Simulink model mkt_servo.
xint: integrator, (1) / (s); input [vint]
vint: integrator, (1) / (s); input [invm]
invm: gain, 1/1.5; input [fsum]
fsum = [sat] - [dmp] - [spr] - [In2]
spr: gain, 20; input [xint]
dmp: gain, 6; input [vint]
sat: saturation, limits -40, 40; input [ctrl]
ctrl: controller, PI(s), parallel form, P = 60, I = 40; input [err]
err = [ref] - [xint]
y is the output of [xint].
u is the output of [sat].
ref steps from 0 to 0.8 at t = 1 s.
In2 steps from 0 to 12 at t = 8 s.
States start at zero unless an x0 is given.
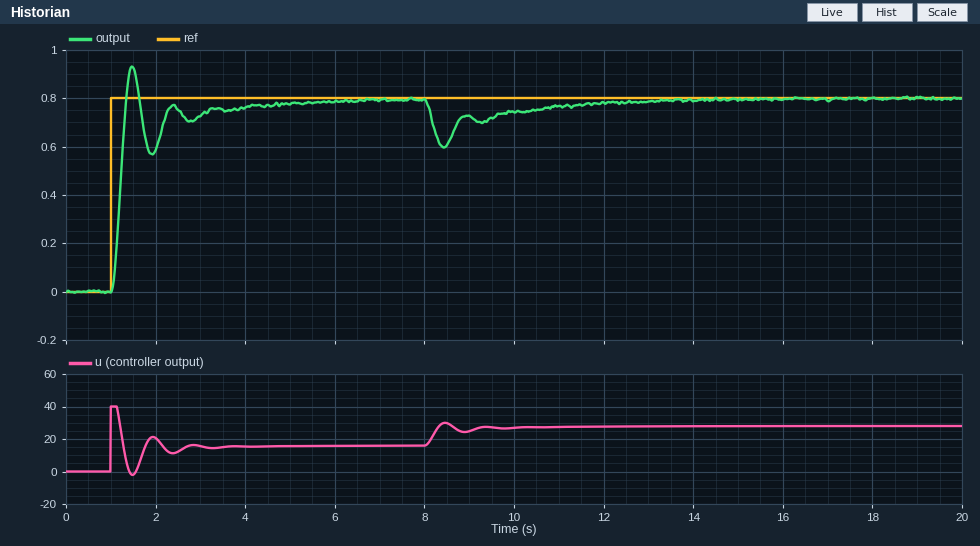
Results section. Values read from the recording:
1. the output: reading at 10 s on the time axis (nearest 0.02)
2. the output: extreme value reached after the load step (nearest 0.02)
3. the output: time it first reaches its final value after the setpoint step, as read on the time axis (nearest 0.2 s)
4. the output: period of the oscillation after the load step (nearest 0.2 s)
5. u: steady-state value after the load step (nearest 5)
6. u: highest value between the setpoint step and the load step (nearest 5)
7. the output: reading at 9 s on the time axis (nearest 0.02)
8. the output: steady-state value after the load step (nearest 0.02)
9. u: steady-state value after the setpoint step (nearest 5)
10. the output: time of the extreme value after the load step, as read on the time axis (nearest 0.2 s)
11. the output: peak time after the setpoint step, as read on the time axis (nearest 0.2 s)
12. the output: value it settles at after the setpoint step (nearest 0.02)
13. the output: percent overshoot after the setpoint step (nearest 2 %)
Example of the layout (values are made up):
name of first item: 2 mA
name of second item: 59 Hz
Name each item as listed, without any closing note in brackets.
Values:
the output: reading at 10 s on the time axis: 0.74
the output: extreme value reached after the load step: 0.60
the output: time it first reaches its final value after the setpoint step, as read on the time axis: 1.4 s
the output: period of the oscillation after the load step: 0.8 s
u: steady-state value after the load step: 30
u: highest value between the setpoint step and the load step: 40
the output: reading at 9 s on the time axis: 0.72
the output: steady-state value after the load step: 0.80
u: steady-state value after the setpoint step: 15
the output: time of the extreme value after the load step, as read on the time axis: 8.4 s
the output: peak time after the setpoint step, as read on the time axis: 1.4 s
the output: value it settles at after the setpoint step: 0.80
the output: percent overshoot after the setpoint step: 16 %
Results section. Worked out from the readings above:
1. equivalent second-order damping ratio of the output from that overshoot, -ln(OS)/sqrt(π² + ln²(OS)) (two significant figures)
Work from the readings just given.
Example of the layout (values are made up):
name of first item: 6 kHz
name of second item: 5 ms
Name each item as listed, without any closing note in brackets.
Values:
equivalent second-order damping ratio of the output from that overshoot, -ln(OS)/sqrt(π² + ln²(OS)): 0.50
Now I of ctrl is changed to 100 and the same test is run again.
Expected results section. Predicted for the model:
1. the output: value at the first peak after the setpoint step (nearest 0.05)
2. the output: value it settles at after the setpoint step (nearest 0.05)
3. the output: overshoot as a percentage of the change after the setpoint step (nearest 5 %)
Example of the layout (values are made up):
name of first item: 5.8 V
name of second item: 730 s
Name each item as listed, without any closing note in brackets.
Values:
the output: value at the first peak after the setpoint step: 1.05
the output: value it settles at after the setpoint step: 0.80
the output: overshoot as a percentage of the change after the setpoint step: 35 %
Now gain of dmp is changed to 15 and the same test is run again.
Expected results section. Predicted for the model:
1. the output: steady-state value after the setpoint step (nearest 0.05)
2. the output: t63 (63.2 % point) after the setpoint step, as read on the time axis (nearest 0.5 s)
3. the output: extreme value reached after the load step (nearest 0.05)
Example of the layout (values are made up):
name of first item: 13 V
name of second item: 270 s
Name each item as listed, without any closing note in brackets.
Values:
the output: steady-state value after the setpoint step: 0.80
the output: t63 (63.2 % point) after the setpoint step, as read on the time axis: 1.5 s
the output: extreme value reached after the load step: 0.65
